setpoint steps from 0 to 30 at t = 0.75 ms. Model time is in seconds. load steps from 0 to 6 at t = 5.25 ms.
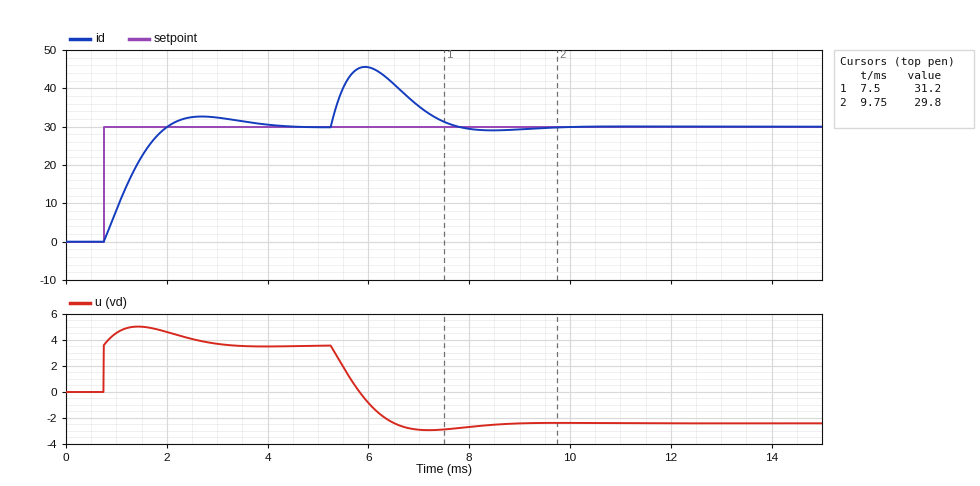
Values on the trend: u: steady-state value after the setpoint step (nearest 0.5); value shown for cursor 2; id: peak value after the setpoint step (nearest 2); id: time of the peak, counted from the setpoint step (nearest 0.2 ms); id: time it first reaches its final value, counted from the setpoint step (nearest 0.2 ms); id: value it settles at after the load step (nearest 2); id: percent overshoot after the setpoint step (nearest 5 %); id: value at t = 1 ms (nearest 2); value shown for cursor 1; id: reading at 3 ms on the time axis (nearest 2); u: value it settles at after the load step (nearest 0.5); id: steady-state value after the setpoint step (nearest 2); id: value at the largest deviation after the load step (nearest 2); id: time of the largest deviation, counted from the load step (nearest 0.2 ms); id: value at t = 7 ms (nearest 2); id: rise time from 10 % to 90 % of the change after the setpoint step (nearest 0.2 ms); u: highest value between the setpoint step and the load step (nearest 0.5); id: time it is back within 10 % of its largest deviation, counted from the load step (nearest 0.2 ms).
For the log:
3.5
29.8
32
2.0 ms
1.2 ms
30
10 %
8
31.2
32
-2.5
30
46
0.6 ms
36
1.0 ms
5.0
2.2 ms
